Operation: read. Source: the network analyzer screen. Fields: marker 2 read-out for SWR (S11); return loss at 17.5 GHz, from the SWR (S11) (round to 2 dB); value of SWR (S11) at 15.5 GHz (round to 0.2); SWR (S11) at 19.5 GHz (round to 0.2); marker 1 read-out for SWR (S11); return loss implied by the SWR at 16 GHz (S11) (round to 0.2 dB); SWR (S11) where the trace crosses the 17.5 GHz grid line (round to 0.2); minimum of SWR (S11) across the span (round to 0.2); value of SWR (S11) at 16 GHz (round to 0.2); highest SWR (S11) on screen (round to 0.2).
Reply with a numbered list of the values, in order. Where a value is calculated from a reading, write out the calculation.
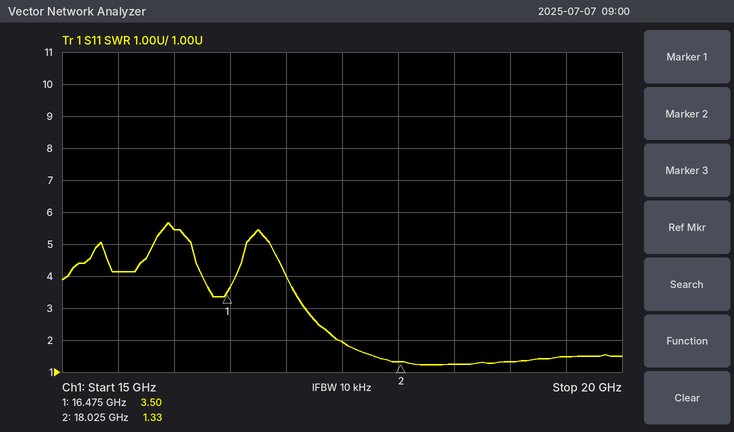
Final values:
1. 1.33
2. −20 log10((2 − 1)/(2 + 1)) ≈ 10 dB
3. 4.2
4. 1.4
5. 3.50
6. −20 log10((5.4 − 1)/(5.4 + 1)) ≈ 3.2 dB
7. 2.0
8. 1.2
9. 5.4
10. 5.6
